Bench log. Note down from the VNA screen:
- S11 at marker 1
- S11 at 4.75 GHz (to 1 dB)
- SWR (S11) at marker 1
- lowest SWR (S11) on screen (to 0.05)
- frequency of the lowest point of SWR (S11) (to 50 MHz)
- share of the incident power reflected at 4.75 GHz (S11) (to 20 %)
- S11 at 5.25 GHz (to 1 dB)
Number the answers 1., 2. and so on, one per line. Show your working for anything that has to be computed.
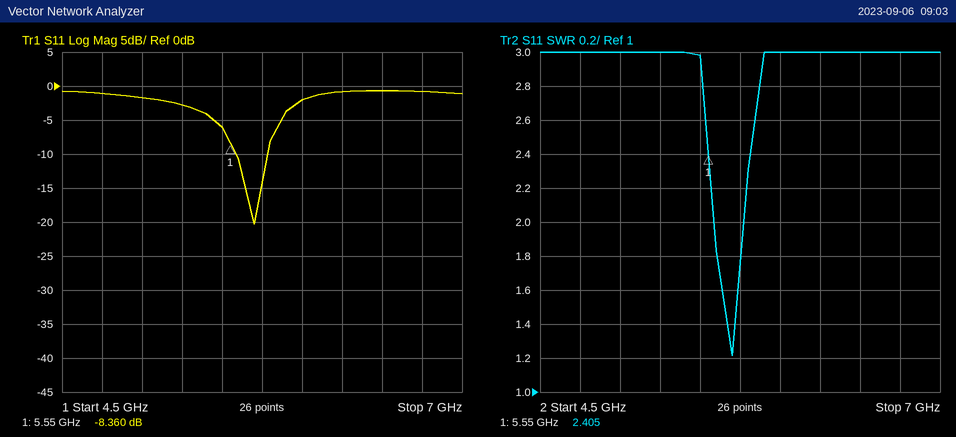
1. -8.360 dB
2. -1 dB
3. 2.405
4. 1.20
5. 5.70 GHz
6. 10^(-1/10) ≈ 79.4 %, so 80 % to the nearest 20 %
7. -3 dB
